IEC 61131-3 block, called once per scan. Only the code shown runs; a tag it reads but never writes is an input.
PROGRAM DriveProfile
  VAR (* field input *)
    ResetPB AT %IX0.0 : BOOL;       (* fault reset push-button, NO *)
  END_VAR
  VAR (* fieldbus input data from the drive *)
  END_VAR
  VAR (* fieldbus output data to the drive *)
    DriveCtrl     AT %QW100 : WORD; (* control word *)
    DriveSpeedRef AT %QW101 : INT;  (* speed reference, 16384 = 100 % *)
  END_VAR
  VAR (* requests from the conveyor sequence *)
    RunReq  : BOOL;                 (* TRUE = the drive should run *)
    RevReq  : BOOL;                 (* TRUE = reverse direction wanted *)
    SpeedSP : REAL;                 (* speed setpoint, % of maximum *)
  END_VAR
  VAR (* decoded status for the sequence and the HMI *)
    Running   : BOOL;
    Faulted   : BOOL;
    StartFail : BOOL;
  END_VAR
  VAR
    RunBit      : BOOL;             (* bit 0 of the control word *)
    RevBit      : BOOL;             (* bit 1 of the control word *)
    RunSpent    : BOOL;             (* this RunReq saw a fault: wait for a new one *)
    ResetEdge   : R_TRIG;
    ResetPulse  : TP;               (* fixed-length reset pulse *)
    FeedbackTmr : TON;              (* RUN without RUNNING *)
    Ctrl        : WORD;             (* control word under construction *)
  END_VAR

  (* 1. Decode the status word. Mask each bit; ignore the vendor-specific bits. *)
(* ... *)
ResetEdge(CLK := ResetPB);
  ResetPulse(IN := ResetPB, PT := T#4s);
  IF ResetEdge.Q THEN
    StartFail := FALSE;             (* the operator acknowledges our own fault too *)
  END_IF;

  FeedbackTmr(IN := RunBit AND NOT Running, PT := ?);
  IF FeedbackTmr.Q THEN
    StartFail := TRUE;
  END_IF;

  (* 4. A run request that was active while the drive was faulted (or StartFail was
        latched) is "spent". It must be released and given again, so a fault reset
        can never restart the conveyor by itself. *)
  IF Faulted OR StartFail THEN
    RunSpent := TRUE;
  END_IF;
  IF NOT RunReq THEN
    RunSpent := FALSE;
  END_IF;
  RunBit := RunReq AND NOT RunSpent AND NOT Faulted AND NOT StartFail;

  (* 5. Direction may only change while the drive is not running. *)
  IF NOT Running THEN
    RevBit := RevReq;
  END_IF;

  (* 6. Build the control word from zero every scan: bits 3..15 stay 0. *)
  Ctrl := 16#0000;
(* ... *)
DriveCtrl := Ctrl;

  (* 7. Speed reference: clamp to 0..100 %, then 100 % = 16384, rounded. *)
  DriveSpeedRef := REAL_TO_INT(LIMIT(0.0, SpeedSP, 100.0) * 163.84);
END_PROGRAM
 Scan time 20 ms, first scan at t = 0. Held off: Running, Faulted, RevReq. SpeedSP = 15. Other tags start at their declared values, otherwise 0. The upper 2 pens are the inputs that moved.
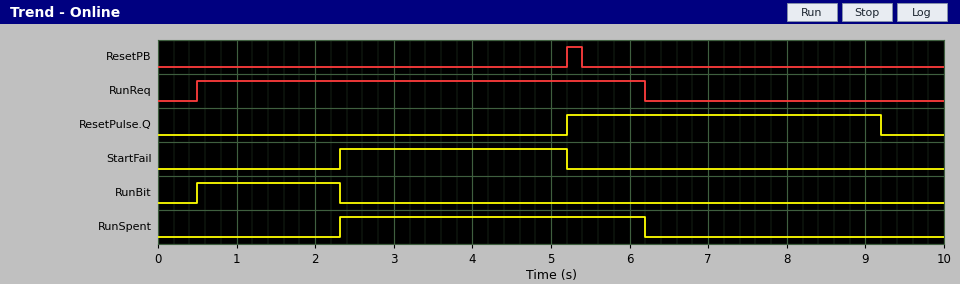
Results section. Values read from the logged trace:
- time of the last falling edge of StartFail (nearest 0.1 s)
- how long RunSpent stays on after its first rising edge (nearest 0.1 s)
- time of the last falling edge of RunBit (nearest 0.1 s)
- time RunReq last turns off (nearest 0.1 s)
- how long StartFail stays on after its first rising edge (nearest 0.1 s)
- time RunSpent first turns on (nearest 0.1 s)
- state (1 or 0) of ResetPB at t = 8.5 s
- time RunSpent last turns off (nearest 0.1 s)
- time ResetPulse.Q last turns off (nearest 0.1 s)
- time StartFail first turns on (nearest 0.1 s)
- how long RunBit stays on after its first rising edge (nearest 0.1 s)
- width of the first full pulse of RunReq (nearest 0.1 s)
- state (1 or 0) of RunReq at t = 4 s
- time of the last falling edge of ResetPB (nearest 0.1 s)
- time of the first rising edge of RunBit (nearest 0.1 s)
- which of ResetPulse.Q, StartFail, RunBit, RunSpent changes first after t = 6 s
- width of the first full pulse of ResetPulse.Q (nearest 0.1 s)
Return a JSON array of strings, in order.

["5.2 s", "3.9 s", "2.3 s", "6.2 s", "2.9 s", "2.3 s", "0", "6.2 s", "9.2 s", "2.3 s", "1.8 s", "5.7 s", "1", "5.4 s", "0.5 s", "RunSpent", "4.0 s"]
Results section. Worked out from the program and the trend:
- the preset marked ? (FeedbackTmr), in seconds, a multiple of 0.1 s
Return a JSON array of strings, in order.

["1.8 s"]
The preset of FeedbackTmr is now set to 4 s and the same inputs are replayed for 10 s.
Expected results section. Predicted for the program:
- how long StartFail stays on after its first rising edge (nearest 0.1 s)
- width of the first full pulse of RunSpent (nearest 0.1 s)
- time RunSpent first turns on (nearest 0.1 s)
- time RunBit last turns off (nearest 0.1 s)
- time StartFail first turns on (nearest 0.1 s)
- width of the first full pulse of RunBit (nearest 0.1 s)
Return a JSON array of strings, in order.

["0.7 s", "1.7 s", "4.5 s", "4.5 s", "4.5 s", "4.0 s"]
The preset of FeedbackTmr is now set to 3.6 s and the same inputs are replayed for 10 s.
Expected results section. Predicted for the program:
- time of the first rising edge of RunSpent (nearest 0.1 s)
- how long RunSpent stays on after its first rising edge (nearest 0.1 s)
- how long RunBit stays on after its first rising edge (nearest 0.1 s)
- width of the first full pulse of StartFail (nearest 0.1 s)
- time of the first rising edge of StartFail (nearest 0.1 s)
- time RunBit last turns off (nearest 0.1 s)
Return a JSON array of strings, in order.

["4.1 s", "2.1 s", "3.6 s", "1.1 s", "4.1 s", "4.1 s"]
